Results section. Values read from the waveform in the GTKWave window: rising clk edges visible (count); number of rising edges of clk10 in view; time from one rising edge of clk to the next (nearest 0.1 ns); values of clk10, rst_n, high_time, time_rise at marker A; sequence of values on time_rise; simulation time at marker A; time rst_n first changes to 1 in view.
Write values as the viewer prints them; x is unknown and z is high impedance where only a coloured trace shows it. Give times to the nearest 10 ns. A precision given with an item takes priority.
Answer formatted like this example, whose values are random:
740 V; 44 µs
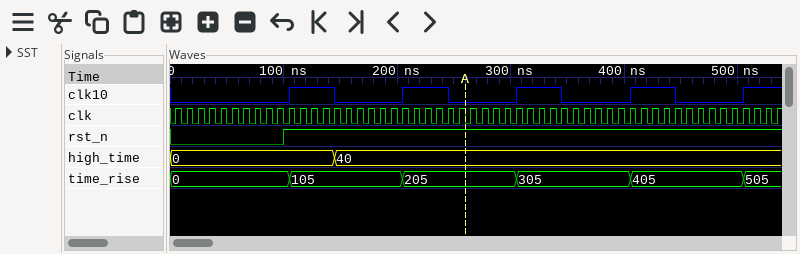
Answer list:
54; 5; 10 ns; clk10=0, rst_n=1, high_time=40, time_rise=205; 0, 105, 205, 305, 405, 505; 260 ns; 100 ns
